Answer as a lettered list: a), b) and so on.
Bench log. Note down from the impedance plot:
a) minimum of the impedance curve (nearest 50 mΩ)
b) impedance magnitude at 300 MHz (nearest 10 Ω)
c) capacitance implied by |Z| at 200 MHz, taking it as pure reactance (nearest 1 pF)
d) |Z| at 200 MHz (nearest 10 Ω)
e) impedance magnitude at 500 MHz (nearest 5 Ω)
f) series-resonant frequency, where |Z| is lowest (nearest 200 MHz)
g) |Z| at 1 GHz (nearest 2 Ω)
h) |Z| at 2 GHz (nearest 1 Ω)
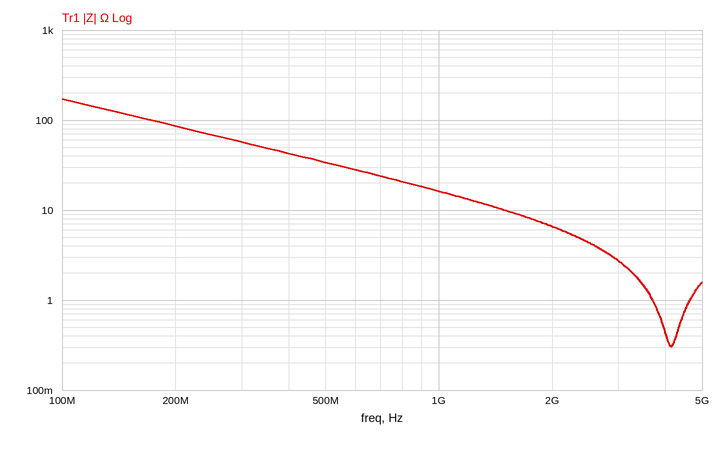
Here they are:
a) 300 mΩ
b) 60 Ω
c) 9 pF
d) 90 Ω
e) 35 Ω
f) 4.2 GHz
g) 16 Ω
h) 7 Ω
